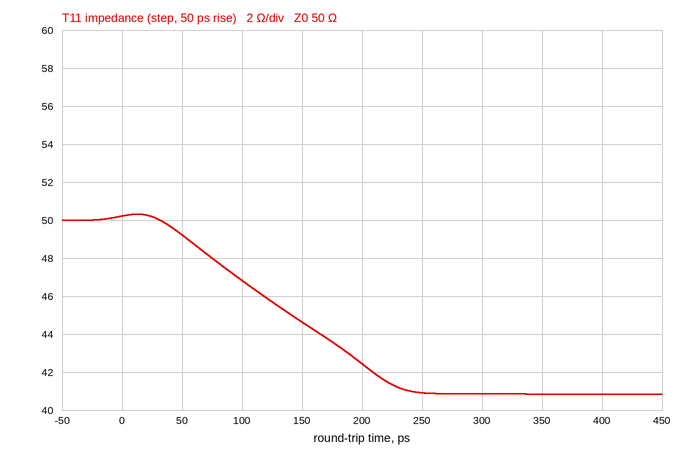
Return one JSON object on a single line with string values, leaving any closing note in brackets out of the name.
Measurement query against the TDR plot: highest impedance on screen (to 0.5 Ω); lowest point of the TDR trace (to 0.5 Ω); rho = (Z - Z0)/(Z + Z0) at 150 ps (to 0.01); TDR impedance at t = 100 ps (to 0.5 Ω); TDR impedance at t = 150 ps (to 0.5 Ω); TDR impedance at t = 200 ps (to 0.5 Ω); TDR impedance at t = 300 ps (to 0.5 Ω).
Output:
{"highest impedance on screen": "50.5 Ω", "lowest point of the TDR trace": "41.0 Ω", "rho = (Z - Z0)/(Z + Z0) at 150 ps": "-0.06", "TDR impedance at t = 100 ps": "47.0 Ω", "TDR impedance at t = 150 ps": "44.5 Ω", "TDR impedance at t = 200 ps": "42.5 Ω", "TDR impedance at t = 300 ps": "41.0 Ω"}
